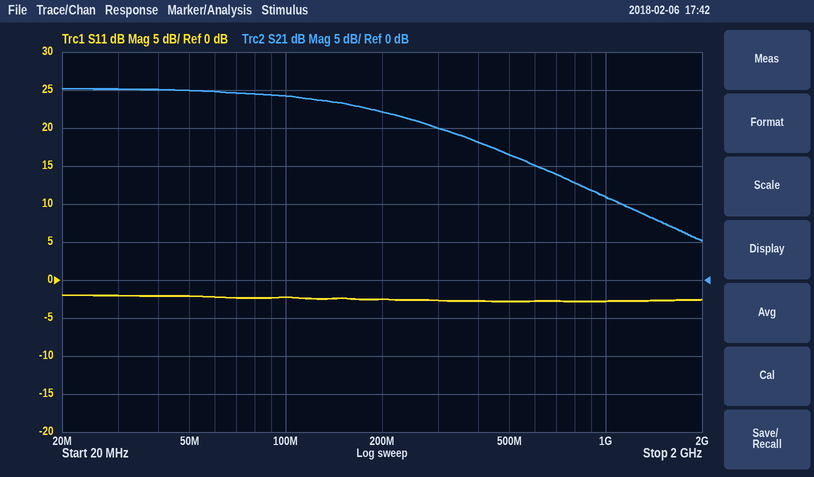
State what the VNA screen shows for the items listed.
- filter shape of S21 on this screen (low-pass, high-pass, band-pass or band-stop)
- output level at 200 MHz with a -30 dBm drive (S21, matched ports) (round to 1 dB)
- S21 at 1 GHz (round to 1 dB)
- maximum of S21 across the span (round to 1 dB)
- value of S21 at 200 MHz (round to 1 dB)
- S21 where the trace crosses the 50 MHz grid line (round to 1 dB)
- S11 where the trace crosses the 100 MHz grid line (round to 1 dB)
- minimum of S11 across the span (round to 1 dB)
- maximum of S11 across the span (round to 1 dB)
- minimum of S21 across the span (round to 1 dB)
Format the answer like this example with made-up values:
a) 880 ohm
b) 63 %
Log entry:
a) low-pass
b) -8 dBm
c) 11 dB
d) 25 dB
e) 22 dB
f) 25 dB
g) -2 dB
h) -3 dB
i) -2 dB
j) 5 dB
